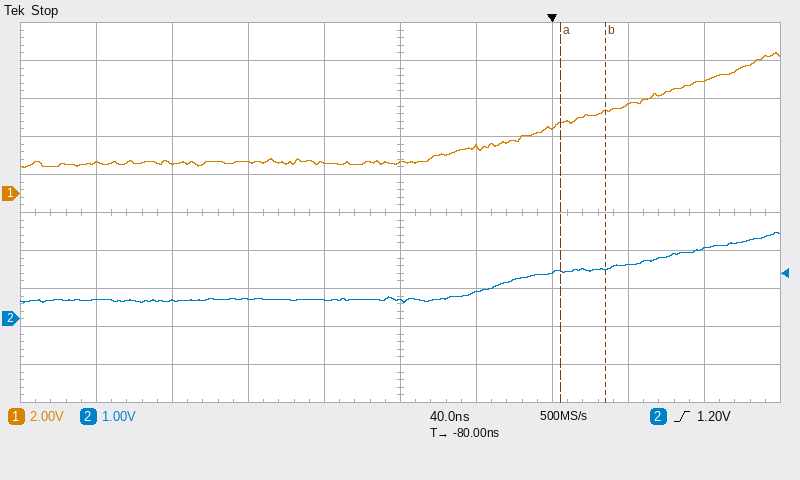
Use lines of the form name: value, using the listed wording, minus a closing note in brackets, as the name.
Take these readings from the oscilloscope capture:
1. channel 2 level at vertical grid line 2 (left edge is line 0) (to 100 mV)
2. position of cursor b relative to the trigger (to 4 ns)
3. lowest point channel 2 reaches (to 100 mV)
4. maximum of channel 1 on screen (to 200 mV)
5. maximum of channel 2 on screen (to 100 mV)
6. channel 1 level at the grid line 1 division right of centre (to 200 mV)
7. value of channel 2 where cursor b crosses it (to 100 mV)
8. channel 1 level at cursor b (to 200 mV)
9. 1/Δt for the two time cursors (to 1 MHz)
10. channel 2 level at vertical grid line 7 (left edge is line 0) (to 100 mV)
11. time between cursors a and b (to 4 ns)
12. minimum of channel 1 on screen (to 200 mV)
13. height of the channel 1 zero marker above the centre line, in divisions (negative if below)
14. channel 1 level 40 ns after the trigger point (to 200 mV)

channel 2 level at vertical grid line 2 (left edge is line 0): 500 mV
position of cursor b relative to the trigger: +28 ns
lowest point channel 2 reaches: 400 mV
maximum of channel 1 on screen: 7.4 V
maximum of channel 2 on screen: 2.3 V
channel 1 level at the grid line 1 division right of centre: 2.4 V
value of channel 2 where cursor b crosses it: 1.3 V
channel 1 level at cursor b: 4.4 V
1/Δt for the two time cursors: 42 MHz
channel 2 level at vertical grid line 7 (left edge is line 0): 1.2 V
time between cursors a and b: 24 ns
minimum of channel 1 on screen: 1.4 V
height of the channel 1 zero marker above the centre line, in divisions: +0.5 div
channel 1 level 40 ns after the trigger point: 4.6 V
